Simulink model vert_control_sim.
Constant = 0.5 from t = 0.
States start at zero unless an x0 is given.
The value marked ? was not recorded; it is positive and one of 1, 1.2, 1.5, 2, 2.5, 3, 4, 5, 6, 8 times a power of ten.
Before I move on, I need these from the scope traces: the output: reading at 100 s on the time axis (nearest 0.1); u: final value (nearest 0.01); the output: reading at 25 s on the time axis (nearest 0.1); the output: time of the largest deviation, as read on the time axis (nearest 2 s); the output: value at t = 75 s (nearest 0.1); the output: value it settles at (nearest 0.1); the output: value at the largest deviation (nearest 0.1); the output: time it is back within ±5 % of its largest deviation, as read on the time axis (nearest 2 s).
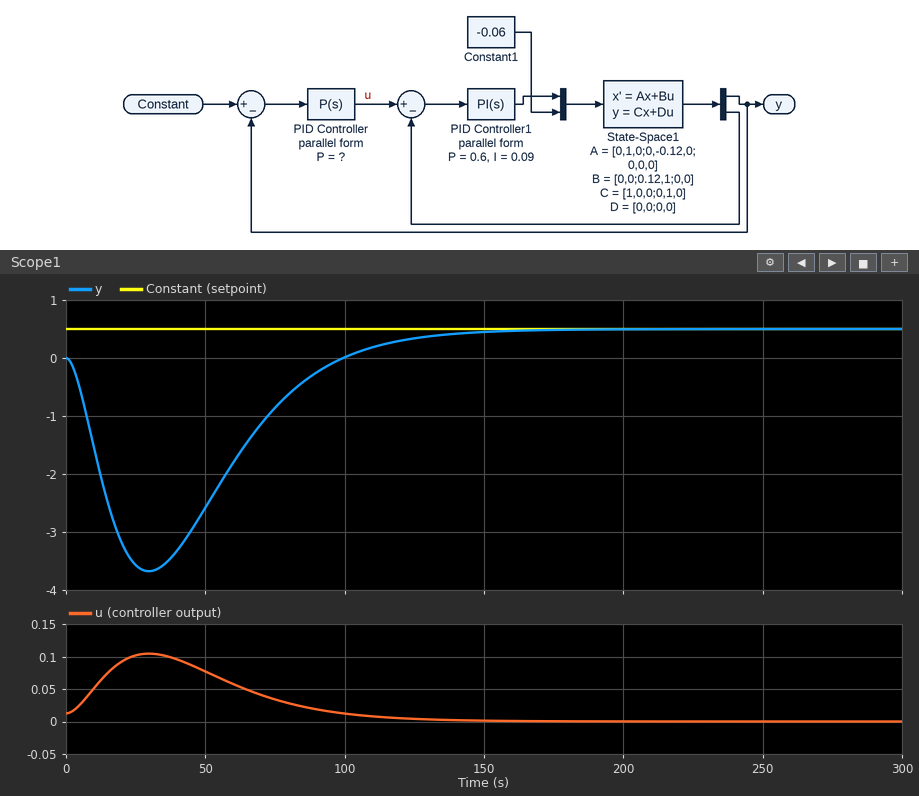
0.0
0.00
-3.6
30 s
-0.9
0.5
-3.7
122 s
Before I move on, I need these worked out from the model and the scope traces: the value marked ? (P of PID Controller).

0.025
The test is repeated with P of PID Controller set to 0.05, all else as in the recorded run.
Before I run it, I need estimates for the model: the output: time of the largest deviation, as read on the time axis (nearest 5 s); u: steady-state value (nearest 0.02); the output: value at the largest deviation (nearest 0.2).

25 s
0.00
-3.0
